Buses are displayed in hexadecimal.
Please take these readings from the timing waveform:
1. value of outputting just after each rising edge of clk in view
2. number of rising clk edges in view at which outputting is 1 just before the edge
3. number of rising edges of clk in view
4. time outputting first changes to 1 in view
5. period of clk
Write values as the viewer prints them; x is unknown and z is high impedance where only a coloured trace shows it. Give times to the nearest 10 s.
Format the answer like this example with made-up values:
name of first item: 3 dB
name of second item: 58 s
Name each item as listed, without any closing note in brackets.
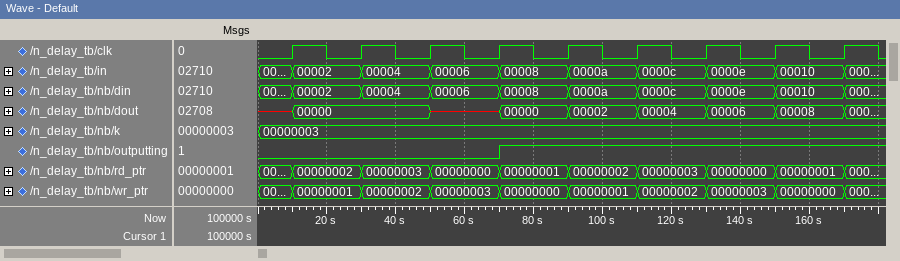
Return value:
value of outputting just after each rising edge of clk in view: 0 0 0 1 1 1 1 1 1
number of rising clk edges in view at which outputting is 1 just before the edge: 5
number of rising edges of clk in view: 9
time outputting first changes to 1 in view: 70 s
period of clk: 20 s
